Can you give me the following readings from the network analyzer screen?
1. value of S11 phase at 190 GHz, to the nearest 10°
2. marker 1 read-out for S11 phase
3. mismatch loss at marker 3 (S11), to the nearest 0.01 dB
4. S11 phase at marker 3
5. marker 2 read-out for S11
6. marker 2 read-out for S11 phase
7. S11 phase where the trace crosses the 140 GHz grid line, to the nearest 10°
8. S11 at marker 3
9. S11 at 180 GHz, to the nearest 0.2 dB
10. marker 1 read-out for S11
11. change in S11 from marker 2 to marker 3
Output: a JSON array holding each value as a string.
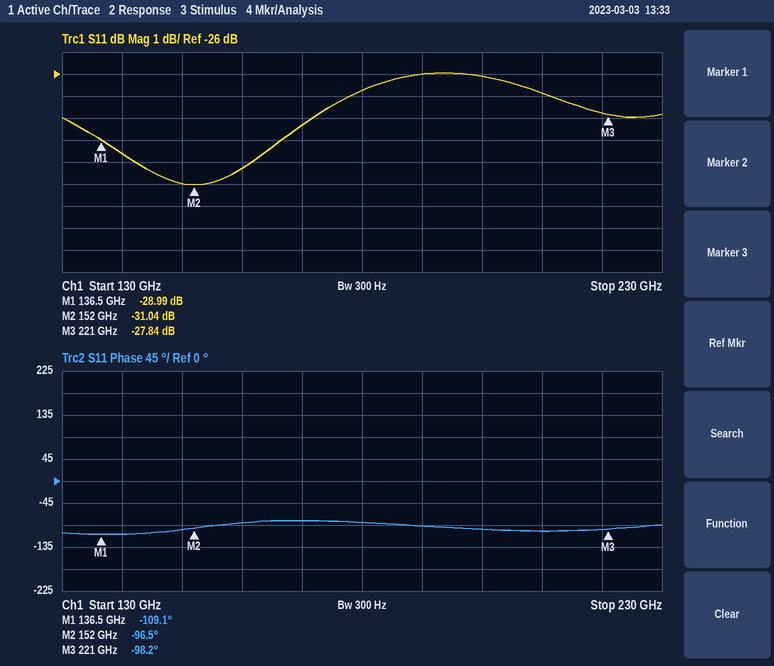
["-90°", "-109.1°", "0.01 dB", "-98.2°", "-31.04 dB", "-96.5°", "-110°", "-27.84 dB", "-26.8 dB", "-28.99 dB", "3.20 dB"]
